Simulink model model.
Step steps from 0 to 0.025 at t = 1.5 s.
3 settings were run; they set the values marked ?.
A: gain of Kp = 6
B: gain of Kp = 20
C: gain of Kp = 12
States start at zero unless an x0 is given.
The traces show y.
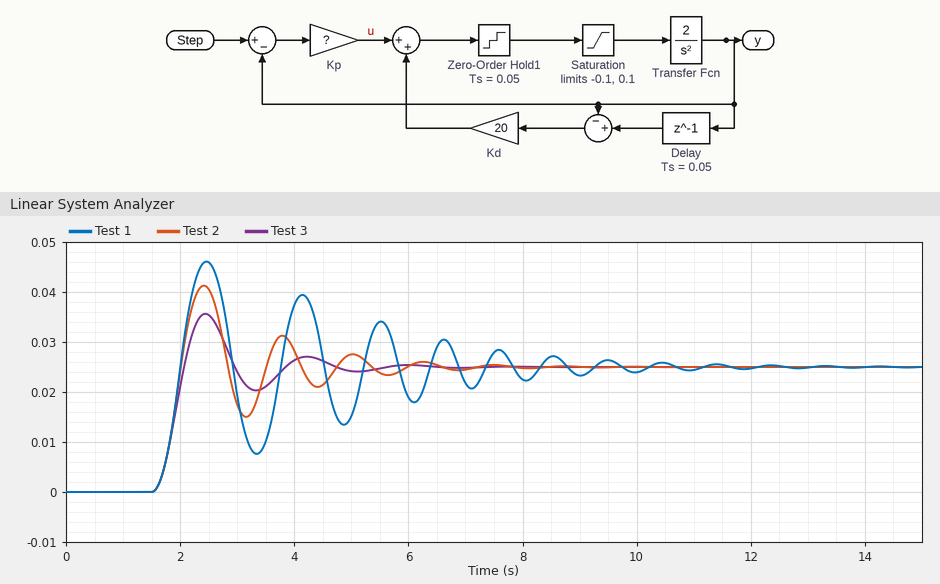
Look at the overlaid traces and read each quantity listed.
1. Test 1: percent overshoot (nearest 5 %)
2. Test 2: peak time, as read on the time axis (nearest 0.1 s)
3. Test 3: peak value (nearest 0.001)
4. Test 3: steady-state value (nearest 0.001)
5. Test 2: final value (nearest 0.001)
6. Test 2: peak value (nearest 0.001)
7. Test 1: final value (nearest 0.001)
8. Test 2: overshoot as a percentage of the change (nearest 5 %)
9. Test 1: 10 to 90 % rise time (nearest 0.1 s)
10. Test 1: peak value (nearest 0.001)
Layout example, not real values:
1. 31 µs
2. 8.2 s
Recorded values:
1. 85 %
2. 2.4 s
3. 0.036
4. 0.025
5. 0.025
6. 0.041
7. 0.025
8. 65 %
9. 0.3 s
10. 0.046
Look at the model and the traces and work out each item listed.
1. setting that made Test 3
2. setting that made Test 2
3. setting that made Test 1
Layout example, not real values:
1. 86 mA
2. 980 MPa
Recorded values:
1. A
2. C
3. B
